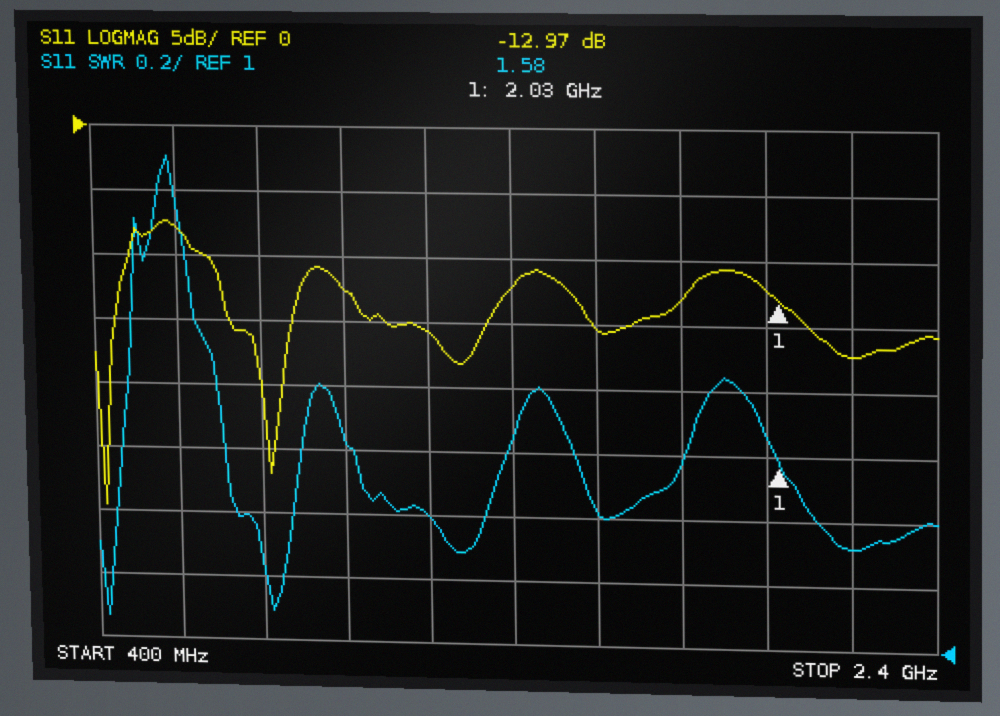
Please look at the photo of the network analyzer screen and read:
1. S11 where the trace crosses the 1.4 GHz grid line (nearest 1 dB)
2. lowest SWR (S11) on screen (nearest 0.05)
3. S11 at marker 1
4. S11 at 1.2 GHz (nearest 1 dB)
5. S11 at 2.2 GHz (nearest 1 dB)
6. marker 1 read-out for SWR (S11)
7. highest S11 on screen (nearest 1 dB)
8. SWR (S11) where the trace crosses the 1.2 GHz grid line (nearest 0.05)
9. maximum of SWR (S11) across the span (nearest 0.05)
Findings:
-12 dB
1.05
-12.97 dB
-16 dB
-17 dB
1.58
-7 dB
1.40
2.50
